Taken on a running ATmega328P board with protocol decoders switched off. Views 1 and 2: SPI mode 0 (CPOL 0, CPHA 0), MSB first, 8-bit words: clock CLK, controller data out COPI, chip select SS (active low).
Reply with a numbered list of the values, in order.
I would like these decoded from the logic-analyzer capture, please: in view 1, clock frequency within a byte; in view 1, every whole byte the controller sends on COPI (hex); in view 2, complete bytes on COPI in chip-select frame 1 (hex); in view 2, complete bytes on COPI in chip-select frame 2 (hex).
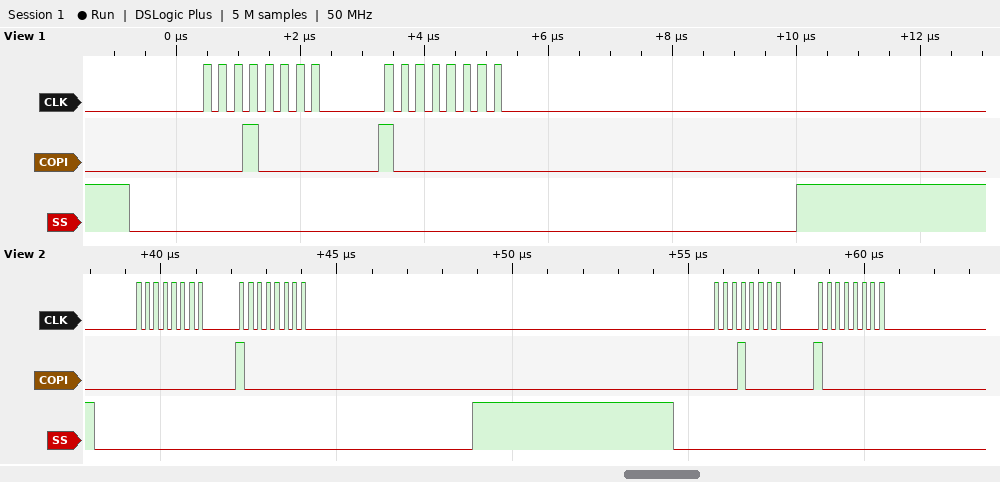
1. 4 MHz
2. 0x10 0x80
3. 0x00 0x80
4. 0x10 0x80
